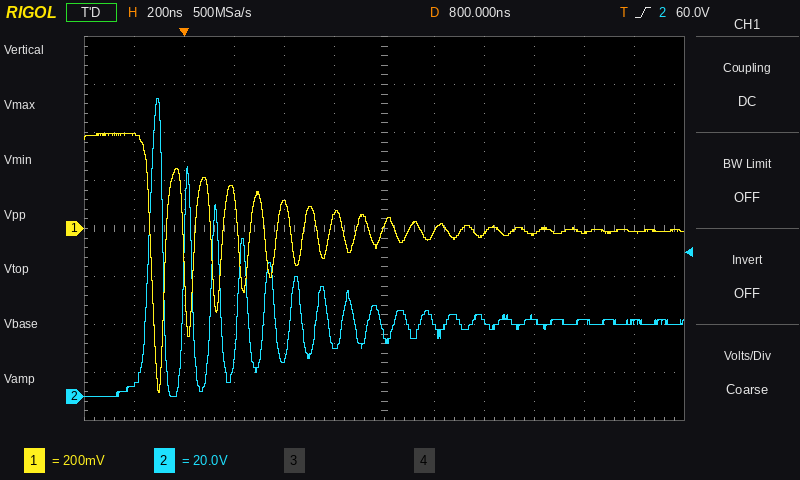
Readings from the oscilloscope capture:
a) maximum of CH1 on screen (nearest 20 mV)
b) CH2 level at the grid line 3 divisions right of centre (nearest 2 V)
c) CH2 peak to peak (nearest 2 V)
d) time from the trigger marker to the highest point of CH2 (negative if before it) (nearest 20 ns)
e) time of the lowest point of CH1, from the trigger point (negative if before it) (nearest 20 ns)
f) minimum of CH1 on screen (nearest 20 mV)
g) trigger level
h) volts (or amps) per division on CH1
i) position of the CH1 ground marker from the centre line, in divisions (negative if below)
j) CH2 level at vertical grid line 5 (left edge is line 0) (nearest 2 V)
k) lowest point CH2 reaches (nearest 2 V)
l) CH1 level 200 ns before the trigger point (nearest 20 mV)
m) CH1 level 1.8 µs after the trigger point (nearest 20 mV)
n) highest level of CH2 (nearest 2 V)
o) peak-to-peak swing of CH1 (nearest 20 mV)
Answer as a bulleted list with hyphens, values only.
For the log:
- 400 mV
- 32 V
- 124 V
- -100 ns
- -100 ns
- -680 mV
- 60.0 V
- 200 mV
- 0.0 div
- 22 V
- 0 V
- 400 mV
- -20 mV
- 124 V
- 1.08 V
